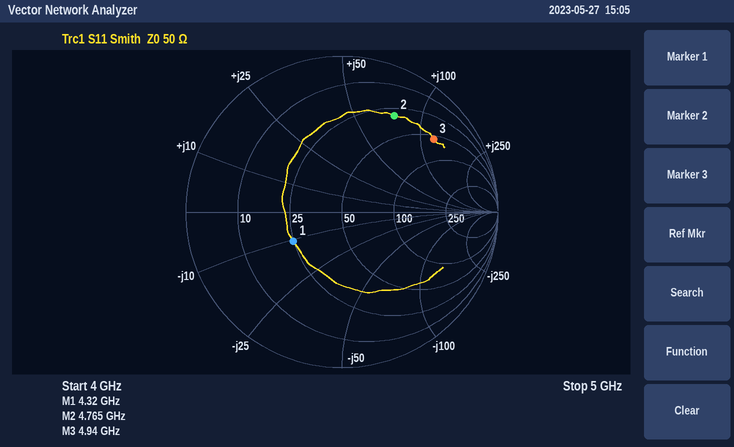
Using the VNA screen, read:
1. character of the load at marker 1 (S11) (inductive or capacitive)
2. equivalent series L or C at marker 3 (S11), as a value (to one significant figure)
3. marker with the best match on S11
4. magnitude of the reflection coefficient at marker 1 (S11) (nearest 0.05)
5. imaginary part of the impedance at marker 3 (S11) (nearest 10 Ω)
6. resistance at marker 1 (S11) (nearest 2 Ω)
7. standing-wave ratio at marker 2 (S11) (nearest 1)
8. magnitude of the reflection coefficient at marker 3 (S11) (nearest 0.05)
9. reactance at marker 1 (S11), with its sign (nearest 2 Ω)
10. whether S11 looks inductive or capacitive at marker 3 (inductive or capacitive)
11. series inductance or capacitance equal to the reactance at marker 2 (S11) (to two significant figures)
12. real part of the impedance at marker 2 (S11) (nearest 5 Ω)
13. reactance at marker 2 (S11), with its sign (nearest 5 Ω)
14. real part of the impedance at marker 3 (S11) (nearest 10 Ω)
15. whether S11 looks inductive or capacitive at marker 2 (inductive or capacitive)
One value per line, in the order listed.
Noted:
capacitive
4 nH
marker 1
0.35
+120 Ω
24 Ω
6
0.75
-10 Ω
inductive
2.5 nH
30 Ω
+75 Ω
60 Ω
inductive
